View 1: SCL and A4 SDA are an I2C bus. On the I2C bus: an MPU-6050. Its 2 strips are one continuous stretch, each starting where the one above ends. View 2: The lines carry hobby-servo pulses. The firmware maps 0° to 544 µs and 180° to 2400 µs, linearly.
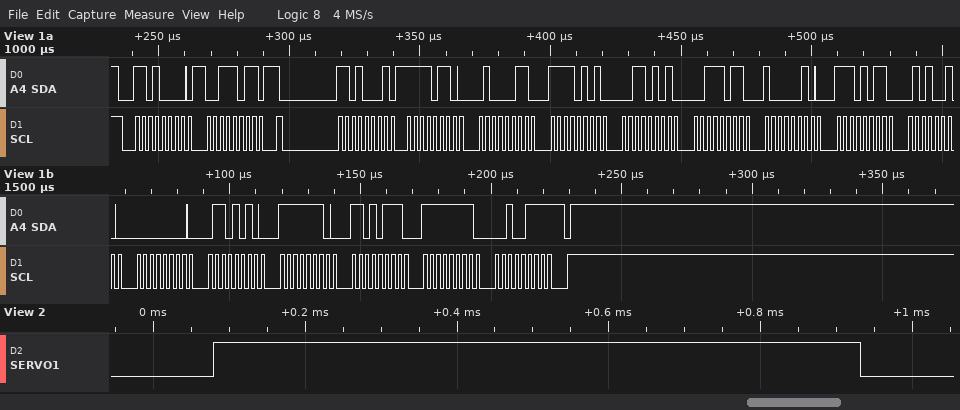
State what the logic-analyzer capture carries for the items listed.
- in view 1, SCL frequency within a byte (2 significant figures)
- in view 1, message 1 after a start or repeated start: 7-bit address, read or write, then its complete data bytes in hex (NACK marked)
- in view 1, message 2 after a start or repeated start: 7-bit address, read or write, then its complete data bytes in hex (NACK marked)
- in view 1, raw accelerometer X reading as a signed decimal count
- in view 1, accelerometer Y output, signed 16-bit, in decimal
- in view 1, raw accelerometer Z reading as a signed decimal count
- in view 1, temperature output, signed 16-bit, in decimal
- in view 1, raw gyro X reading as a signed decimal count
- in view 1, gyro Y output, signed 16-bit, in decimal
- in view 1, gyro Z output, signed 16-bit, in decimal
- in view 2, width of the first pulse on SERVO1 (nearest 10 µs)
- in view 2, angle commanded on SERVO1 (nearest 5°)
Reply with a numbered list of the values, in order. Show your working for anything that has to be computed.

1. 400 kHz
2. 0x68 write: 3B
3. 0x68 read: F6 43 F5 35 3B 82 EB 52 00 6A FE D7 FF 27 NACK
4. 0xF643 = -2493
5. 0xF535 = -2763
6. 0x3B82 = 15234
7. 0xEB52 = -5294
8. 0x006A = 106
9. 0xFED7 = -297
10. 0xFF27 = -217
11. 850 µs
12. 30°
